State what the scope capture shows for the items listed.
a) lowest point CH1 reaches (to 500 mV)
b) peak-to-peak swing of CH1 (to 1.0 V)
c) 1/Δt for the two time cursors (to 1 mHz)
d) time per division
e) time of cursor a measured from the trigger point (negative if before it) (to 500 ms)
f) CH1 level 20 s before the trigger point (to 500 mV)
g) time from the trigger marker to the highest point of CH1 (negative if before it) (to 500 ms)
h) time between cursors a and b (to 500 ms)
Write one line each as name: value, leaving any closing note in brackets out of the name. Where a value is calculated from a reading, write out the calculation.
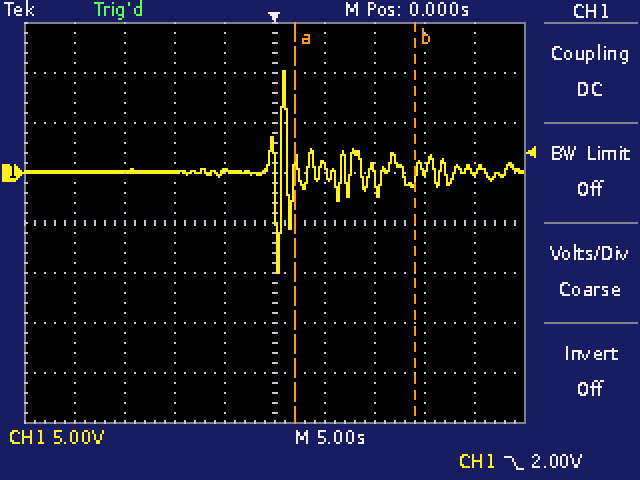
lowest point CH1 reaches: -10.0 V
peak-to-peak swing of CH1: 20.0 V
1/Δt for the two time cursors: 1 / 12.0 s ≈ 83 mHz
time per division: 5 s
time of cursor a measured from the trigger point (negative if before it): +2.0 s
CH1 level 20 s before the trigger point: 0.0 V
time from the trigger marker to the highest point of CH1 (negative if before it): +1.0 s
time between cursors a and b: 12.0 s
